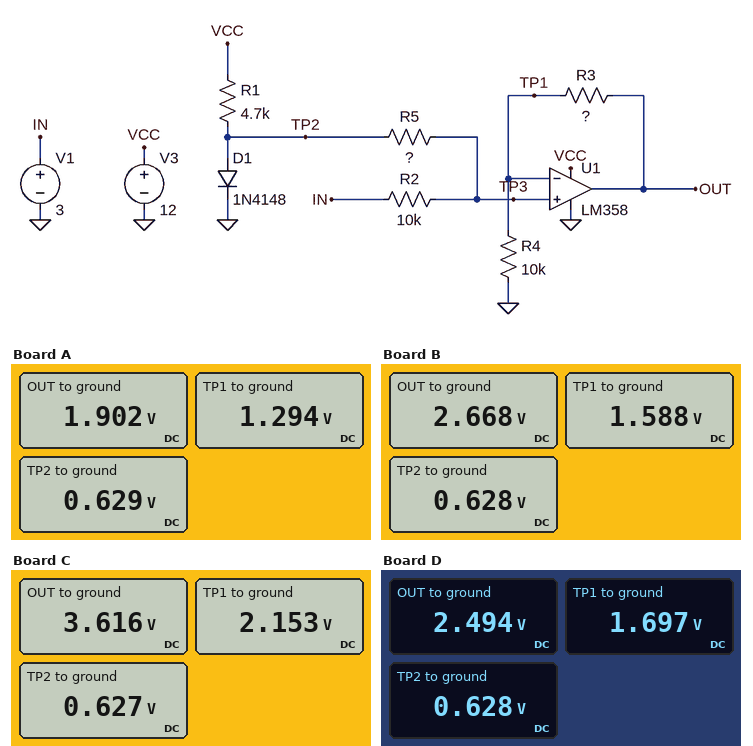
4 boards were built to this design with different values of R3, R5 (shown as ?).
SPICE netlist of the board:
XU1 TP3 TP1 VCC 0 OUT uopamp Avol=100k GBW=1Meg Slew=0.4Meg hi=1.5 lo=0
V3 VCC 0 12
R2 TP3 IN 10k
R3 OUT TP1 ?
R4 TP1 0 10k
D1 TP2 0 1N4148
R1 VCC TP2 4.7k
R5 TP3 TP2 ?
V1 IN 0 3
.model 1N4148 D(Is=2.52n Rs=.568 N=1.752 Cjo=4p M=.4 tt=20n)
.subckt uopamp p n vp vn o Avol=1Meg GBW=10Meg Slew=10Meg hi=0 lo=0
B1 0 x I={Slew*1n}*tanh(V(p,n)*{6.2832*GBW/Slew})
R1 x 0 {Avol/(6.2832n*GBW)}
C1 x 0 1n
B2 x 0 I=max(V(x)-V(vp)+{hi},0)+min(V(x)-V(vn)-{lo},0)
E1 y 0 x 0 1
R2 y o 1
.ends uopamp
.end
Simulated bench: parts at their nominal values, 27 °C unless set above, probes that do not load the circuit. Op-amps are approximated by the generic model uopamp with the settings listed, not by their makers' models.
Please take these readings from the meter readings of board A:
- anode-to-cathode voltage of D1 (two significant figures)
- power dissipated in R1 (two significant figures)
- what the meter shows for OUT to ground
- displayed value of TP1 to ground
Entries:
630 mV
28 mW
1.902 V
1.294 V
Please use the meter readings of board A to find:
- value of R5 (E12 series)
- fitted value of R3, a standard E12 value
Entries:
3.9 kΩ
4.7 kΩ
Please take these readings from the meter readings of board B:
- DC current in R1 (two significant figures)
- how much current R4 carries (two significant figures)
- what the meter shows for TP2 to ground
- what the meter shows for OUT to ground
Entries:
2.4 mA
160 µA
0.628 V
2.668 V
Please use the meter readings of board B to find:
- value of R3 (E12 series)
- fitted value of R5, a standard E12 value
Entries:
6.8 kΩ
6.8 kΩ
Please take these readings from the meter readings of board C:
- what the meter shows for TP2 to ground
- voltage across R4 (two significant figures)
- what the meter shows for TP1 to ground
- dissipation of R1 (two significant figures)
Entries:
0.627 V
2.2 V
2.153 V
28 mW
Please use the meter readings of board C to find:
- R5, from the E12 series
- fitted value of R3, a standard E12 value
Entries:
18 kΩ
6.8 kΩ
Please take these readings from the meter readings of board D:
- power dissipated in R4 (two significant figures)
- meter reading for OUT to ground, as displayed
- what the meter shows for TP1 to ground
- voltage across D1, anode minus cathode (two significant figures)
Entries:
290 µW
2.494 V
1.697 V
630 mV
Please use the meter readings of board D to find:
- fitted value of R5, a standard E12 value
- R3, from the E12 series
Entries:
8.2 kΩ
4.7 kΩ
